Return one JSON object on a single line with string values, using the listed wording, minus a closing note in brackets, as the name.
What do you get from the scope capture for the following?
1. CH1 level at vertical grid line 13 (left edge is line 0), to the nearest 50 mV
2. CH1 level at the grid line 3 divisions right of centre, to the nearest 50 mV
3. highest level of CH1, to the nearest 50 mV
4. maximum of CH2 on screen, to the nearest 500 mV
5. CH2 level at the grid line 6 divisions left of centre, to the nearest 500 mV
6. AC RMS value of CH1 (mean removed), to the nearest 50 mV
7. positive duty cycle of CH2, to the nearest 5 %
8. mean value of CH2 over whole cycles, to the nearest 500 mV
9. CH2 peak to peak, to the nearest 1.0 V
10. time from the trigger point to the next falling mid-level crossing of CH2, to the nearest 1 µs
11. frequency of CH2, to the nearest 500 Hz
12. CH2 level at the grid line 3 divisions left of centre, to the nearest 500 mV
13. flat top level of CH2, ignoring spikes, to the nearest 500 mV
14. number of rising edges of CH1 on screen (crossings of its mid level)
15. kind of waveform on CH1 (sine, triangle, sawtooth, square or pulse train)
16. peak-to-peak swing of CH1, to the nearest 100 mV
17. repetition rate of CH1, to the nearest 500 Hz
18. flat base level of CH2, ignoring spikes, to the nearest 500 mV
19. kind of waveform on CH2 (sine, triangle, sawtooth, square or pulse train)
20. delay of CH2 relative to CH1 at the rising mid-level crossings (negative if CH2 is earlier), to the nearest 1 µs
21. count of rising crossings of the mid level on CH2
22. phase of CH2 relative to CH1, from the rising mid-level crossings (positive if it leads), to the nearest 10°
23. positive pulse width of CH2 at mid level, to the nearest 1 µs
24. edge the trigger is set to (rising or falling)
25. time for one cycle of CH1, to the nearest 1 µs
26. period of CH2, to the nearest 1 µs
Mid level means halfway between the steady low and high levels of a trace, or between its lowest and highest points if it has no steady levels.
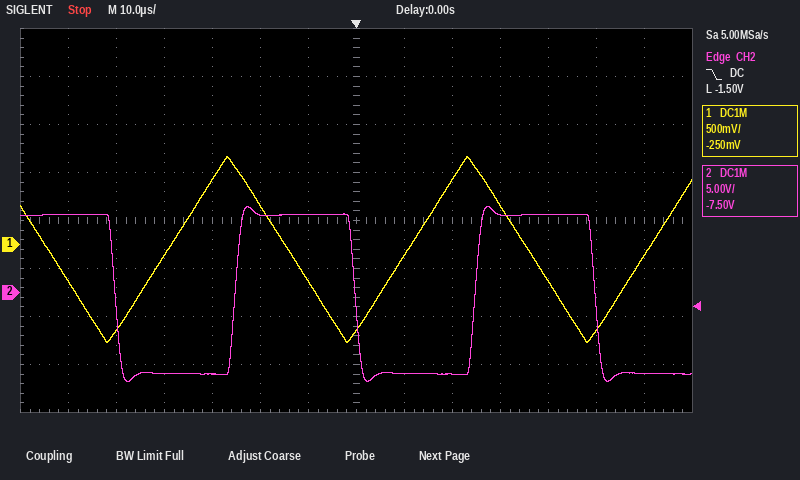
{"CH1 level at vertical grid line 13 (left edge is line 0), to the nearest 50 mV": "-100 mV", "CH1 level at the grid line 3 divisions right of centre, to the nearest 50 mV": "400 mV", "highest level of CH1, to the nearest 50 mV": "900 mV", "maximum of CH2 on screen, to the nearest 500 mV": "9.0 V", "CH2 level at the grid line 6 divisions left of centre, to the nearest 500 mV": "8.0 V", "AC RMS value of CH1 (mean removed), to the nearest 50 mV": "550 mV", "positive duty cycle of CH2, to the nearest 5 %": "50 %", "mean value of CH2 over whole cycles, to the nearest 500 mV": "0.0 V", "CH2 peak to peak, to the nearest 1.0 V": "18.0 V", "time from the trigger point to the next falling mid-level crossing of CH2, to the nearest 1 µs": "50 µs", "frequency of CH2, to the nearest 500 Hz": "20.0 kHz", "CH2 level at the grid line 3 divisions left of centre, to the nearest 500 mV": "-8.5 V", "flat top level of CH2, ignoring spikes, to the nearest 500 mV": "8.0 V", "number of rising edges of CH1 on screen": "3", "kind of waveform on CH1": "triangle", "peak-to-peak swing of CH1, to the nearest 100 mV": "1.90 V", "repetition rate of CH1, to the nearest 500 Hz": "20.0 kHz", "flat base level of CH2, ignoring spikes, to the nearest 500 mV": "-8.5 V", "kind of waveform on CH2": "square", "delay of CH2 relative to CH1 at the rising mid-level crossings (negative if CH2 is earlier), to the nearest 1 µs": "+14 µs", "count of rising crossings of the mid level on CH2": "2", "phase of CH2 relative to CH1, from the rising mid-level crossings (positive if it leads), to the nearest 10°": "-100°", "positive pulse width of CH2 at mid level, to the nearest 1 µs": "25 µs", "edge the trigger is set to": "falling", "time for one cycle of CH1, to the nearest 1 µs": "50 µs", "period of CH2, to the nearest 1 µs": "50 µs"}
